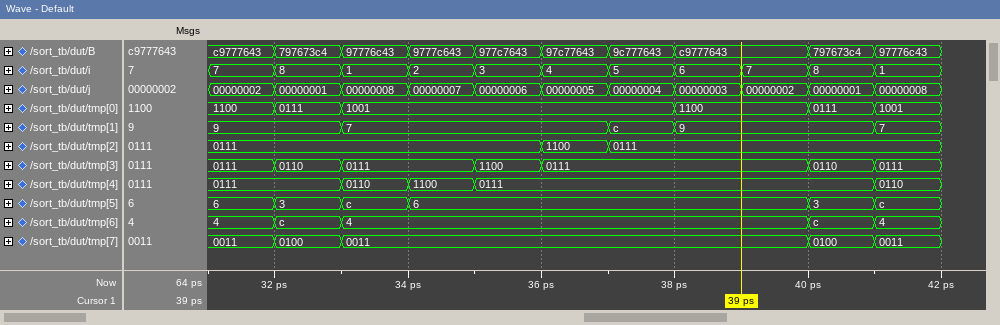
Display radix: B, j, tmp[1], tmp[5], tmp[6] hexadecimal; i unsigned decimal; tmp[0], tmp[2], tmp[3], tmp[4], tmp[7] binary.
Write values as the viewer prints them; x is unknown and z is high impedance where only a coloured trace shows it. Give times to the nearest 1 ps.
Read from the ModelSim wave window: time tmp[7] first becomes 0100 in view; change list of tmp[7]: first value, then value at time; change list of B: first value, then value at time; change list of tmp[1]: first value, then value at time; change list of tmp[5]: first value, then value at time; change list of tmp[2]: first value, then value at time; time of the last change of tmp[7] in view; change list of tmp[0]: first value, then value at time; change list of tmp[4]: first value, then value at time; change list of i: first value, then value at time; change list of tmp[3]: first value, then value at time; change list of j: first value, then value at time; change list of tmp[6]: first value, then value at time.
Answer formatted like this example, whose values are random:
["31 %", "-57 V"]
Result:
["32 ps", "0011, 0100 at 32 ps, 0011 at 33 ps, 0100 at 40 ps, 0011 at 41 ps", "c9777643, 797673c4 at 32 ps, 97776c43 at 33 ps, 9777c643 at 34 ps, 977c7643 at 35 ps, 97c77643 at 36 ps, 9c777643 at 37 ps, c9777643 at 38 ps, 797673c4 at 40 ps, 97776c43 at 41 ps", "9, 7 at 33 ps, c at 37 ps, 9 at 38 ps, 7 at 41 ps", "6, 3 at 32 ps, c at 33 ps, 6 at 34 ps, 3 at 40 ps, c at 41 ps", "0111, 1100 at 36 ps, 0111 at 37 ps", "41 ps", "1100, 0111 at 32 ps, 1001 at 33 ps, 1100 at 38 ps, 0111 at 40 ps, 1001 at 41 ps", "0111, 0110 at 33 ps, 1100 at 34 ps, 0111 at 35 ps, 0110 at 41 ps", "7, 8 at 32 ps, 1 at 33 ps, 2 at 34 ps, 3 at 35 ps, 4 at 36 ps, 5 at 37 ps, 6 at 38 ps, 7 at 39 ps, 8 at 40 ps, 1 at 41 ps", "0111, 0110 at 32 ps, 0111 at 33 ps, 1100 at 35 ps, 0111 at 36 ps, 0110 at 40 ps, 0111 at 41 ps", "00000002, 00000001 at 32 ps, 00000008 at 33 ps, 00000007 at 34 ps, 00000006 at 35 ps, 00000005 at 36 ps, 00000004 at 37 ps, 00000003 at 38 ps, 00000002 at 39 ps, 00000001 at 40 ps, 00000008 at 41 ps", "4, c at 32 ps, 4 at 33 ps, c at 40 ps, 4 at 41 ps"]
